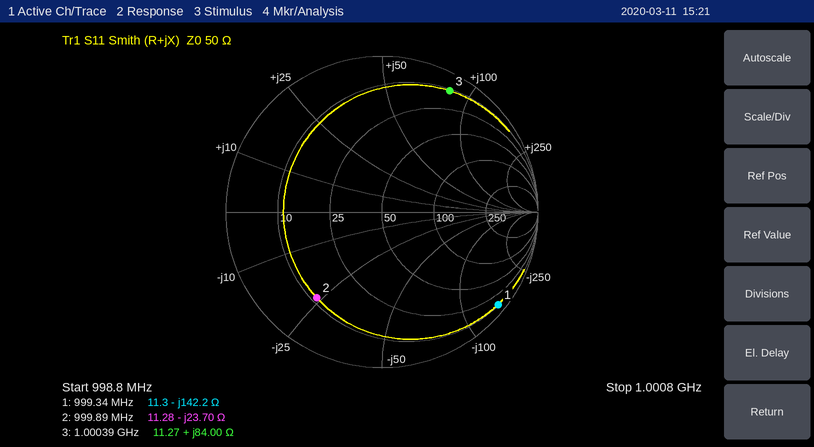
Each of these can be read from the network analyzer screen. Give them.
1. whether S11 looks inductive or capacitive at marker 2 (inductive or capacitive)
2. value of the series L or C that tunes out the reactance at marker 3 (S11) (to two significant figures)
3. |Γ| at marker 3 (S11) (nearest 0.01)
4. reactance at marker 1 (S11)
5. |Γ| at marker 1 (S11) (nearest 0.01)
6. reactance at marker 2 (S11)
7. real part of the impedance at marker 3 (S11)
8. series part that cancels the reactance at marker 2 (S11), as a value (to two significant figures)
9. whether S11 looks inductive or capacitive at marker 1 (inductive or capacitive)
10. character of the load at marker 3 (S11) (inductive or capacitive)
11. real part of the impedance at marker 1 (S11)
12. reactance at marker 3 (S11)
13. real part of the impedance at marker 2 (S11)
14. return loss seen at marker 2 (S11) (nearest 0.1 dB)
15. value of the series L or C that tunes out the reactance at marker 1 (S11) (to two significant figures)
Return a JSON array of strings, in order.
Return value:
["capacitive", "1.9 pF", "0.89", "-142.2 Ω", "0.95", "-23.70 Ω", "11.27 Ω", "3.8 nH", "capacitive", "inductive", "11.3 Ω", "+84.00 Ω", "11.28 Ω", "3.2 dB", "23 nH"]
